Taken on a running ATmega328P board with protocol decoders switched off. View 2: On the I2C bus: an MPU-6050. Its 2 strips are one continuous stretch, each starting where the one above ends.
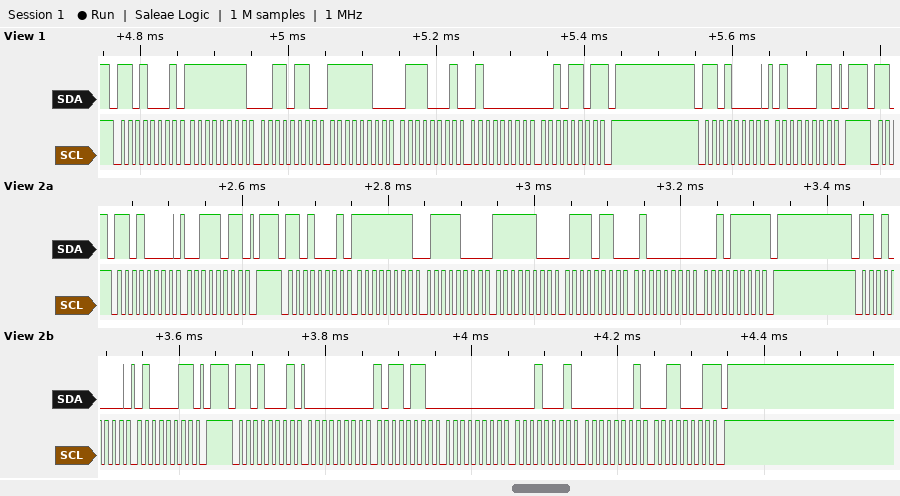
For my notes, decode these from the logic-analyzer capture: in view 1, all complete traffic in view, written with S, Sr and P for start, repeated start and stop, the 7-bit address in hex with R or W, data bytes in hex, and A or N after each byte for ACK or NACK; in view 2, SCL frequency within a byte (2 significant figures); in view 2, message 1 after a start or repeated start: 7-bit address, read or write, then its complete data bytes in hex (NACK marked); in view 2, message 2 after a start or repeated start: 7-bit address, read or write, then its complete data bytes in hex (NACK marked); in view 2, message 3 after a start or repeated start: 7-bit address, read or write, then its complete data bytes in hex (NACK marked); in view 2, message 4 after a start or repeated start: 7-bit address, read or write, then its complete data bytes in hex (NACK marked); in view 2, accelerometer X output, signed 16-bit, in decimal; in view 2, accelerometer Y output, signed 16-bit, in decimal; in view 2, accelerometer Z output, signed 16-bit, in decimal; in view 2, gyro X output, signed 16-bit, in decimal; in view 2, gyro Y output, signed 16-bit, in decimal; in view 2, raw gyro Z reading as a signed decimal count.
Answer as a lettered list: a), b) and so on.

a) S 68R A FF A 36 A FC A 71 A 40 A 2D N P S 68W A 43 A P
b) 100 kHz
c) 0x68 write: 3B
d) 0x68 read: FF 78 FC 76 40 2F NACK
e) 0x68 write: 43
f) 0x68 read: 00 B6 00 11 01 31 NACK
g) -136
h) -906
i) 16431
j) 182
k) 17
l) 305
